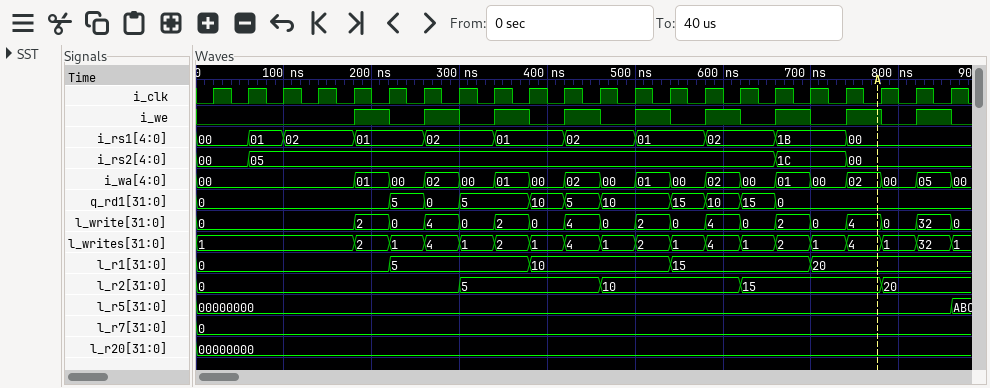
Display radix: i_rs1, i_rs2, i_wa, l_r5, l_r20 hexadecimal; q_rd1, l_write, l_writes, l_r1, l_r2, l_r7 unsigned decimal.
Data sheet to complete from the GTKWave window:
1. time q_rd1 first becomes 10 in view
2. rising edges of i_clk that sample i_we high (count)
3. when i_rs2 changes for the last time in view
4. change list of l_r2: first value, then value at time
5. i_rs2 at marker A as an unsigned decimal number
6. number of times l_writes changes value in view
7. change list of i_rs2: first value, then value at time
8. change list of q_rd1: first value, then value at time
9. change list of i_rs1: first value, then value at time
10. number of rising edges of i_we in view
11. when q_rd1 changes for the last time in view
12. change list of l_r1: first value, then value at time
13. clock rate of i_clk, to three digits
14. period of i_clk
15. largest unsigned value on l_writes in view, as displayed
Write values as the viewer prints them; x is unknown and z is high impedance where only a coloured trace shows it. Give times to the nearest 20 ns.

380 ns
9
740 ns
0, 5 at 300 ns, 10 at 460 ns, 15 at 620 ns, 20 at 780 ns
0
18
00, 05 at 60 ns, 1C at 660 ns, 00 at 740 ns
0, 5 at 220 ns, 0 at 260 ns, 5 at 300 ns, 10 at 380 ns, 5 at 420 ns, 10 at 460 ns, 15 at 540 ns, 10 at 580 ns, 15 at 620 ns, 0 at 660 ns
00, 01 at 60 ns, 02 at 100 ns, 01 at 180 ns, 02 at 260 ns, 01 at 340 ns, 02 at 420 ns, 01 at 500 ns, 02 at 580 ns, 1B at 660 ns, 00 at 740 ns
9
660 ns
0, 5 at 220 ns, 10 at 380 ns, 15 at 540 ns, 20 at 700 ns
25.0 MHz
40 ns
32
